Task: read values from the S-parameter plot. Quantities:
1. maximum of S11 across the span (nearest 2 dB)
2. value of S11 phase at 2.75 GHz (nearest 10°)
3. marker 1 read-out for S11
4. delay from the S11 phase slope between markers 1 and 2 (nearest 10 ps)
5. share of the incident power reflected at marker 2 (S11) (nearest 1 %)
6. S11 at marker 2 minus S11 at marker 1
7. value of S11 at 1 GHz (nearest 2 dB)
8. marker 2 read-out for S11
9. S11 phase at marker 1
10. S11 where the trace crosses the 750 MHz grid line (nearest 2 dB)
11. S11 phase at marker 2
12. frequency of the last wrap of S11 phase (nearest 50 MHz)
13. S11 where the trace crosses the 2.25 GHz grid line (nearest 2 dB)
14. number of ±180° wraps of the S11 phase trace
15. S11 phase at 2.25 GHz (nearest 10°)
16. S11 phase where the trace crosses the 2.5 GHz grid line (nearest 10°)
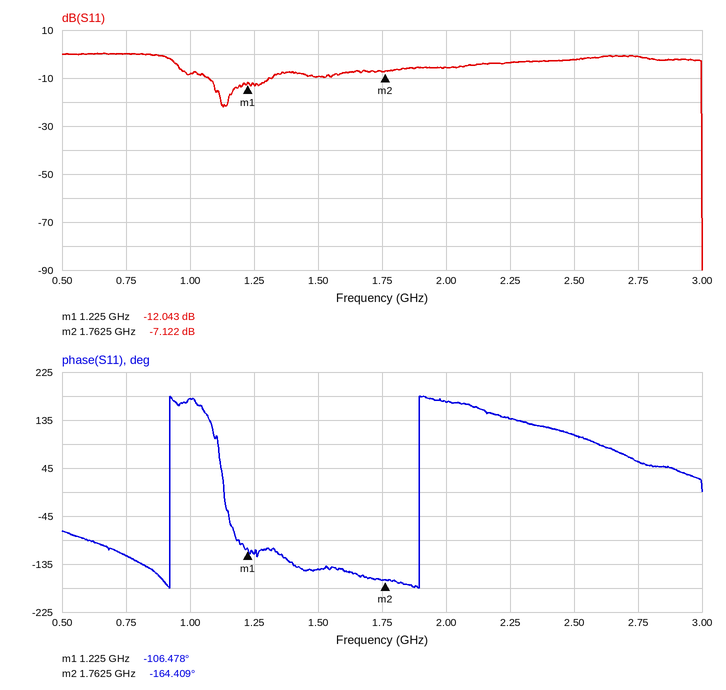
0 dB
60°
-12.043 dB
300 ps
19 %
4.921 dB
-8 dB
-7.122 dB
-106.478°
0 dB
-164.409°
1.90 GHz
-4 dB
2
140°
110°
